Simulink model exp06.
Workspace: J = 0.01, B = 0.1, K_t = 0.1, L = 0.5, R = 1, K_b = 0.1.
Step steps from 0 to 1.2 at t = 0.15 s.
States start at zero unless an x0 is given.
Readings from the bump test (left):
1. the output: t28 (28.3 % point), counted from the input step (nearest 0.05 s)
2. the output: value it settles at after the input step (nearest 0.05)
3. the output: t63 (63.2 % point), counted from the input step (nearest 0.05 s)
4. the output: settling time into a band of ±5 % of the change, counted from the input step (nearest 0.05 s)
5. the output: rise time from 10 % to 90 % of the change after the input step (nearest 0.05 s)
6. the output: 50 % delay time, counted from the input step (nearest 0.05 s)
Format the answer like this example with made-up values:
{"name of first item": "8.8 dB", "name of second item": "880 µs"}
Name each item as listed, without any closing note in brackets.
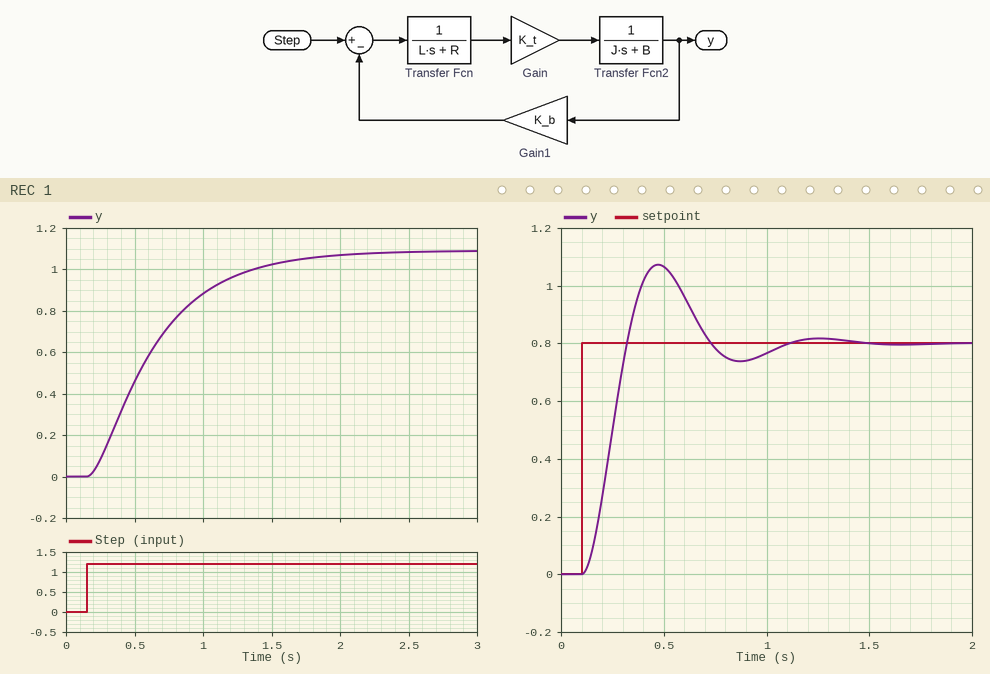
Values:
{"the output: t28 (28.3 % point), counted from the input step": "0.25 s", "the output: value it settles at after the input step": "1.10", "the output: t63 (63.2 % point), counted from the input step": "0.55 s", "the output: settling time into a band of ±5 % of the change, counted from the input step": "1.45 s", "the output: rise time from 10 % to 90 % of the change after the input step": "1.00 s", "the output: 50 % delay time, counted from the input step": "0.40 s"}
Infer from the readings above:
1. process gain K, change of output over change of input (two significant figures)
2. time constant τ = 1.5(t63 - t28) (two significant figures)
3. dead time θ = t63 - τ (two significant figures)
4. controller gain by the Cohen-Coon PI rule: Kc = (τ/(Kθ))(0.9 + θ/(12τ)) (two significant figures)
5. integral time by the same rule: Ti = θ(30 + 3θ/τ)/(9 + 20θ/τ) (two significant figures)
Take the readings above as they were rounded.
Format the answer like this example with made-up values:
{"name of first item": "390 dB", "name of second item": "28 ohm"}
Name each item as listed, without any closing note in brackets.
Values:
{"process gain K, change of output over change of input": "0.92", "time constant τ = 1.5(t63 - t28)": "0.45 s", "dead time θ = t63 - τ": "0.10 s", "controller gain by the Cohen-Coon PI rule: Kc = (τ/(Kθ))(0.9 + θ/(12τ))": "4.5", "integral time by the same rule: Ti = θ(30 + 3θ/τ)/(9 + 20θ/τ)": "0.23 s"}
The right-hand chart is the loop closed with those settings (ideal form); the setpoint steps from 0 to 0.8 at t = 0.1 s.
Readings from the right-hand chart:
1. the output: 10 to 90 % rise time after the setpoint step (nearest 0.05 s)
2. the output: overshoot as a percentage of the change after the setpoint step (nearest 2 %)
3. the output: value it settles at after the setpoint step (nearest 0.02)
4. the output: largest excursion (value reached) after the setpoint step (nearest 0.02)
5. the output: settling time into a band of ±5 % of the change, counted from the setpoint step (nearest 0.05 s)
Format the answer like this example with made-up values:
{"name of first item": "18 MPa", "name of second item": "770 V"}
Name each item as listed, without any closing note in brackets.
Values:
{"the output: 10 to 90 % rise time after the setpoint step": "0.15 s", "the output: overshoot as a percentage of the change after the setpoint step": "34 %", "the output: value it settles at after the setpoint step": "0.80", "the output: largest excursion (value reached) after the setpoint step": "1.08", "the output: settling time into a band of ±5 % of the change, counted from the setpoint step": "0.90 s"}
